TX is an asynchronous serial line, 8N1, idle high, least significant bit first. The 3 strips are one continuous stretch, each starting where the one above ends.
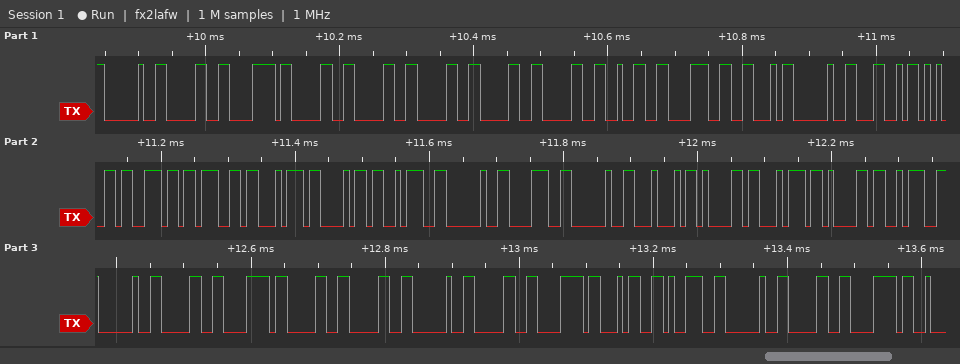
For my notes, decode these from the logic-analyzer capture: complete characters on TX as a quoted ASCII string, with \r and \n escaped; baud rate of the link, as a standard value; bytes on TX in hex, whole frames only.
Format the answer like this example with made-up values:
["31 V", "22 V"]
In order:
["\" 0x0000028F Length: 8 Data: 0x00 0x49 0x\"", "115200 baud", "20 30 78 30 30 30 30 30 32 38 46 20 4C 65 6E 67 74 68 3A 20 38 20 44 61 74 61 3A 20 30 78 30 30 20 30 78 34 39 20 30 78"]
